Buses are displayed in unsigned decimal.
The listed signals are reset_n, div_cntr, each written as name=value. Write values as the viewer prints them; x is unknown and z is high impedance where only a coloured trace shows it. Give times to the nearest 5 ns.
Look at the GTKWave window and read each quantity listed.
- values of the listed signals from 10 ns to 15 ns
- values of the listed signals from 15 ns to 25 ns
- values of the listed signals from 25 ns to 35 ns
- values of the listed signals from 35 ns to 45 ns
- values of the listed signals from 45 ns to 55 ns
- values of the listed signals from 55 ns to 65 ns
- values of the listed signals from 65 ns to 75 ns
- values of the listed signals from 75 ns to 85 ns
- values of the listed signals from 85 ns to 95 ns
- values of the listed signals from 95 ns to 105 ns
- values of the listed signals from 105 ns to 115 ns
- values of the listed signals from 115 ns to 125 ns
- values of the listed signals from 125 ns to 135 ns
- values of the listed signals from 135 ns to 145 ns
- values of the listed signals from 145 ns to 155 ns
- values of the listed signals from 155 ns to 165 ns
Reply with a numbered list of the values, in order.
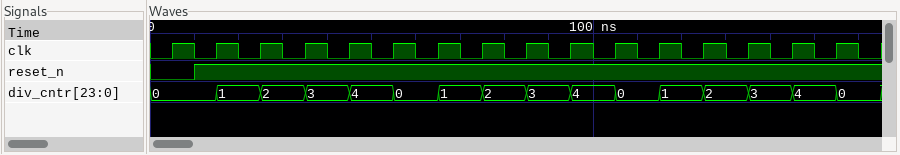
1. reset_n=1, div_cntr=0
2. reset_n=1, div_cntr=1
3. reset_n=1, div_cntr=2
4. reset_n=1, div_cntr=3
5. reset_n=1, div_cntr=4
6. reset_n=1, div_cntr=0
7. reset_n=1, div_cntr=1
8. reset_n=1, div_cntr=2
9. reset_n=1, div_cntr=3
10. reset_n=1, div_cntr=4
11. reset_n=1, div_cntr=0
12. reset_n=1, div_cntr=1
13. reset_n=1, div_cntr=2
14. reset_n=1, div_cntr=3
15. reset_n=1, div_cntr=4
16. reset_n=1, div_cntr=0
